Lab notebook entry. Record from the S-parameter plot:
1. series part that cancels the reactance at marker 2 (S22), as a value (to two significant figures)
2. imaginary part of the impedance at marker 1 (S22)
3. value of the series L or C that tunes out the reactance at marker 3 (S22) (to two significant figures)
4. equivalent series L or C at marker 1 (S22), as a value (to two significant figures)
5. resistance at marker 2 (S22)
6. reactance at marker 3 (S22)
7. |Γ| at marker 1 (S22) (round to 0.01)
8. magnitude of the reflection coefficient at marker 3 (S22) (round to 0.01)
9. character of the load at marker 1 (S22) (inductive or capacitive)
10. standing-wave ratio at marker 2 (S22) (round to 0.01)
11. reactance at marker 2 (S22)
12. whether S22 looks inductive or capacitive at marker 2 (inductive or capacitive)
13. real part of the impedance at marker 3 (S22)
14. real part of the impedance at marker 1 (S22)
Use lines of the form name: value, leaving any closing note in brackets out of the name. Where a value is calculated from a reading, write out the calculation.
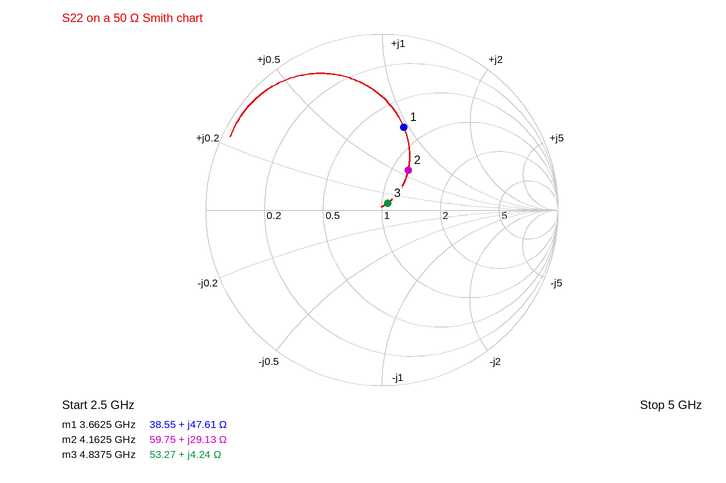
series part that cancels the reactance at marker 2 (S22), as a value: C = 1/(2π × 4.1625 GHz × 29.13 Ω) ≈ 1.3 pF
imaginary part of the impedance at marker 1: +47.61 Ω
value of the series L or C that tunes out the reactance at marker 3 (S22): C = 1/(2π × 4.8375 GHz × 4.24 Ω) ≈ 7.8 pF
equivalent series L or C at marker 1 (S22), as a value: L = 47.61 Ω/(2π × 3.6625 GHz) ≈ 2.1 nH
resistance at marker 2: 59.75 Ω
reactance at marker 3: +4.24 Ω
|Γ| at marker 1 (S22): 0.49
magnitude of the reflection coefficient at marker 3 (S22): 0.05
character of the load at marker 1 (S22): inductive
standing-wave ratio at marker 2 (S22): 1.74
reactance at marker 2: +29.13 Ω
whether S22 looks inductive or capacitive at marker 2: inductive
real part of the impedance at marker 3: 53.27 Ω
real part of the impedance at marker 1: 38.55 Ω
